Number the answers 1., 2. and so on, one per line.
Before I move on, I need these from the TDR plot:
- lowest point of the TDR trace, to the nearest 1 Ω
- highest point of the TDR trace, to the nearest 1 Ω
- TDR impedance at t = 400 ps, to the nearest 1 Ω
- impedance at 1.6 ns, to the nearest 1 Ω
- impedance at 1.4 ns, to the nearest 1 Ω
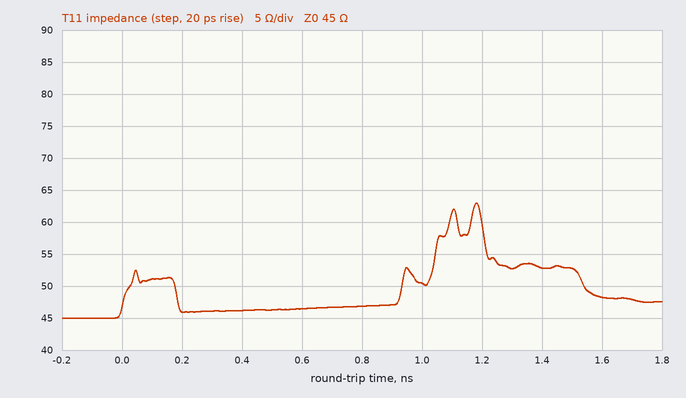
1. 45 Ω
2. 63 Ω
3. 46 Ω
4. 48 Ω
5. 53 Ω
